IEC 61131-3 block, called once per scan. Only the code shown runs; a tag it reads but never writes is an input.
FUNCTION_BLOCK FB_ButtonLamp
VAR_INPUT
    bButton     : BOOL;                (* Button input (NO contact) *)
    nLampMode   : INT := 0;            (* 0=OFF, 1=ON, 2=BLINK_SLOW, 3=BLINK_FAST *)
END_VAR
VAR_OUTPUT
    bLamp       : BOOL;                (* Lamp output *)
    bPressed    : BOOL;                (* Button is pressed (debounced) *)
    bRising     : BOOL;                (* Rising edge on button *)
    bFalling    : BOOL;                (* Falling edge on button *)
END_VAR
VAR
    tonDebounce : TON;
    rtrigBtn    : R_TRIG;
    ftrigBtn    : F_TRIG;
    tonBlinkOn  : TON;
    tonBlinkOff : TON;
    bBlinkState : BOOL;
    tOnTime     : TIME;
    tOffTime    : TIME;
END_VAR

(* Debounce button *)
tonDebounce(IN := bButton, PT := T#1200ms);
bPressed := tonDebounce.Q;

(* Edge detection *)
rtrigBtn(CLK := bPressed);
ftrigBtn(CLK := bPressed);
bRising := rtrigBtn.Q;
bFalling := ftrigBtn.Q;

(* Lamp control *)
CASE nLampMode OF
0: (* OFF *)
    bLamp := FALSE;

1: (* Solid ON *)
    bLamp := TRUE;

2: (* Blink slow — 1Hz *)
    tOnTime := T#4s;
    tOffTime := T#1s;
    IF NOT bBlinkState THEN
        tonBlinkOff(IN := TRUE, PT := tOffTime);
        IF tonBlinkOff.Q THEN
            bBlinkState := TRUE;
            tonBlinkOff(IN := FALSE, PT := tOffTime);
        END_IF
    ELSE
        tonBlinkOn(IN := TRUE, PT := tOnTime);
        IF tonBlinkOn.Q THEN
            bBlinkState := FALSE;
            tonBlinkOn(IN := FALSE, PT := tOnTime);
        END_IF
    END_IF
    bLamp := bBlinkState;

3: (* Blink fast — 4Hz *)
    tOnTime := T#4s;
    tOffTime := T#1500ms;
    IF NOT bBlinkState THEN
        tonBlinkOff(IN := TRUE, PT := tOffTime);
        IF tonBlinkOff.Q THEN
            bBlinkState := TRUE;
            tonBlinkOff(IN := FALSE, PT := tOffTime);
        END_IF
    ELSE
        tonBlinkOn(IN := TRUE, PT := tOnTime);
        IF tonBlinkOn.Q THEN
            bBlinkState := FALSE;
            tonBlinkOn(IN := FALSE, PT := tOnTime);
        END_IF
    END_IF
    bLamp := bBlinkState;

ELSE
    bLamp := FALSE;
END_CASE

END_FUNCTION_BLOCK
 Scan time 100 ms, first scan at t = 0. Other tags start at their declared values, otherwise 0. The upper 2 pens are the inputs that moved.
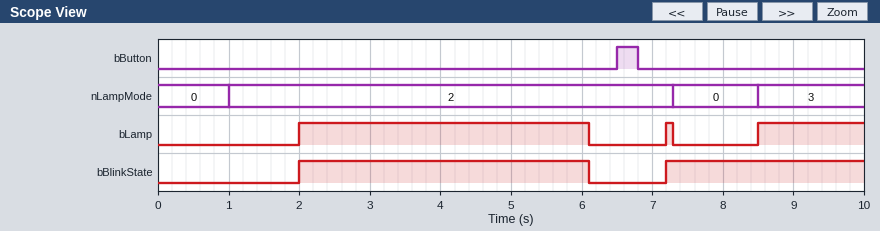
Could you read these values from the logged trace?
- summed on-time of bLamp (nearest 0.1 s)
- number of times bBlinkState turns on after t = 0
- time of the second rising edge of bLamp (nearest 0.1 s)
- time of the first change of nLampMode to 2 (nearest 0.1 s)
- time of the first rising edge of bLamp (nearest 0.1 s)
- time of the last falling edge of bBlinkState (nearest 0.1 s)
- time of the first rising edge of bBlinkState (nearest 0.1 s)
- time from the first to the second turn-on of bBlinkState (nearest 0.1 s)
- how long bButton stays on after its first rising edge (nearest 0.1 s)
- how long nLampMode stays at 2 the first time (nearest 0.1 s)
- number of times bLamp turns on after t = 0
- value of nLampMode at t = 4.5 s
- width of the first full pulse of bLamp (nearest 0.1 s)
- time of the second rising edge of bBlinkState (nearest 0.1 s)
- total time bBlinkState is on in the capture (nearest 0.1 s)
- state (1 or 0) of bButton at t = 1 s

5.7 s
2
7.2 s
1.0 s
2.0 s
6.1 s
2.0 s
5.2 s
0.3 s
6.3 s
3
2
4.1 s
7.2 s
6.9 s
0
